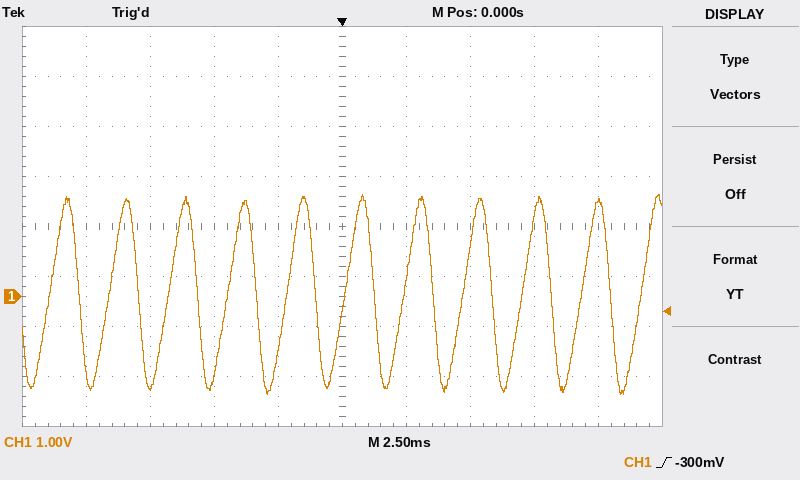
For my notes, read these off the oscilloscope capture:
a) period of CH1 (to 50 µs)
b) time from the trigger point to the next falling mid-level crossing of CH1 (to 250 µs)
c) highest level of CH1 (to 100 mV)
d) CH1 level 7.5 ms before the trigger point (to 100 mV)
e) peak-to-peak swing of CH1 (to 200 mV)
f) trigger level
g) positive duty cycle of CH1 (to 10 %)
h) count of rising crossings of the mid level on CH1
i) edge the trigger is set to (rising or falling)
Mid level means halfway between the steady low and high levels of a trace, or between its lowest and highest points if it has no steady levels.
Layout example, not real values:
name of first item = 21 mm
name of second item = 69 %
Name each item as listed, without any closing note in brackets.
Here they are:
period of CH1 = 2.30 ms
time from the trigger point to the next falling mid-level crossing of CH1 = 1.25 ms
highest level of CH1 = 2.0 V
CH1 level 7.5 ms before the trigger point = -1.8 V
peak-to-peak swing of CH1 = 4.0 V
trigger level = -300 mV
positive duty cycle of CH1 = 50 %
count of rising crossings of the mid level on CH1 = 11
edge the trigger is set to = rising
